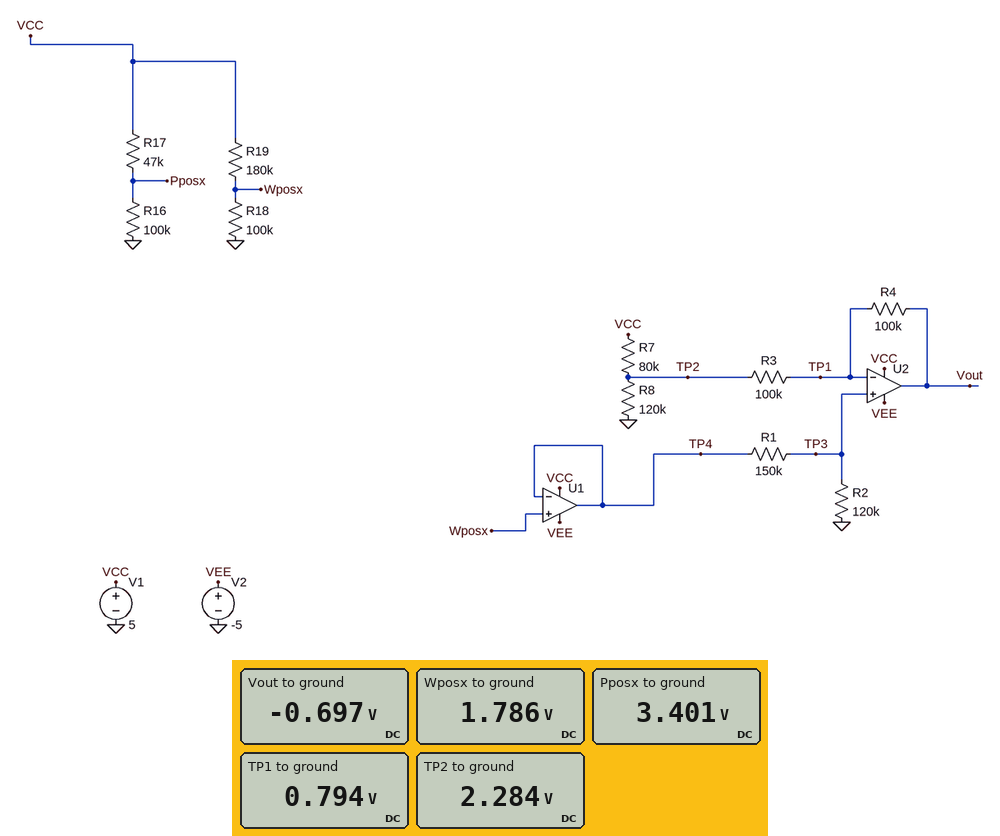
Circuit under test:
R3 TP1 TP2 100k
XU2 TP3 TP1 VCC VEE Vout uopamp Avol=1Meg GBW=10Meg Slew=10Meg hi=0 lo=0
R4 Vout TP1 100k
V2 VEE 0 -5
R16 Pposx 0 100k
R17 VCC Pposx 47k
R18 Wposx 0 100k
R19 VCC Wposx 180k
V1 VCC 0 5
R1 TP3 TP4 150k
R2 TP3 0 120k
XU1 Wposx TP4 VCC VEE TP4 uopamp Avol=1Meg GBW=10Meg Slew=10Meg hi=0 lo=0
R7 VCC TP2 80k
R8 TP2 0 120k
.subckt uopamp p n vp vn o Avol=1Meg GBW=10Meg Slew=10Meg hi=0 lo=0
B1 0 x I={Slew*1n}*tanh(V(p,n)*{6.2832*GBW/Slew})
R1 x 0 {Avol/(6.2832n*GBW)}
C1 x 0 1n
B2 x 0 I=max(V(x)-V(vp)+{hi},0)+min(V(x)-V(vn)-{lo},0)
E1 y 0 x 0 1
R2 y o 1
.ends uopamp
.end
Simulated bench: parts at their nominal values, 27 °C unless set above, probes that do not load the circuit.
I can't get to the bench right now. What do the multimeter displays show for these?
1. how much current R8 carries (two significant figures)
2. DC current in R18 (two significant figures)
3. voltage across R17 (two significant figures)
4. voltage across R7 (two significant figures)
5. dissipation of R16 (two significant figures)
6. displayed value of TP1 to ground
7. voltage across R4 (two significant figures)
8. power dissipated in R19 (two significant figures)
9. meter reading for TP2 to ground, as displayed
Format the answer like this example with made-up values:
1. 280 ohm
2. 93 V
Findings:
1. 19 µA
2. 18 µA
3. 1.6 V
4. 2.7 V
5. 120 µW
6. 0.794 V
7. 1.5 V
8. 57 µW
9. 2.284 V
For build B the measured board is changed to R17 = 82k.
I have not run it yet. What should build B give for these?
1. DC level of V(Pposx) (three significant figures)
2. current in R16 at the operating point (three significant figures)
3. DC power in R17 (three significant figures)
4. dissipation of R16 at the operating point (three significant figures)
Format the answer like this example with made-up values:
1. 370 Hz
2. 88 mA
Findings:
1. 2.75 V
2. 27.5 µA
3. 61.9 µW
4. 75.5 µW
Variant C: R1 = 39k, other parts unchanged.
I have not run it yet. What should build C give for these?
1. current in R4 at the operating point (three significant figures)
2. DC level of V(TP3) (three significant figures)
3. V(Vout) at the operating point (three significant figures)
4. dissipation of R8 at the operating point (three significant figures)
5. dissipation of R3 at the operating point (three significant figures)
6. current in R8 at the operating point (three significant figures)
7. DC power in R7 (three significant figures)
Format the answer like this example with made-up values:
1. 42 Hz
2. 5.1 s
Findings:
1. 11.2 µA
2. 1.35 V
3. 231 mV
4. 50.6 µW
5. 12.5 µW
6. 20.5 µA
7. 80.4 µW
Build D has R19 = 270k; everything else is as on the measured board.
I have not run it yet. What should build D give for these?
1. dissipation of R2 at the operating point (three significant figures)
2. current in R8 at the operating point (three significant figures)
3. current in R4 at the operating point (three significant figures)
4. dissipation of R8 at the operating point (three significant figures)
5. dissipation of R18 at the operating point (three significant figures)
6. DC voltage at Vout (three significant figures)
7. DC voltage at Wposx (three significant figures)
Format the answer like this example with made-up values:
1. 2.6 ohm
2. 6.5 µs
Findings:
1. 3.01 µW
2. 18.5 µA
3. 16.2 µA
4. 41.1 µW
5. 18.3 µW
6. -1.02 V
7. 1.35 V
